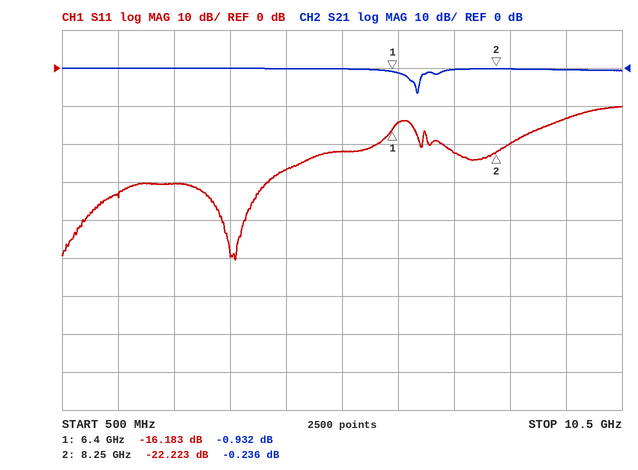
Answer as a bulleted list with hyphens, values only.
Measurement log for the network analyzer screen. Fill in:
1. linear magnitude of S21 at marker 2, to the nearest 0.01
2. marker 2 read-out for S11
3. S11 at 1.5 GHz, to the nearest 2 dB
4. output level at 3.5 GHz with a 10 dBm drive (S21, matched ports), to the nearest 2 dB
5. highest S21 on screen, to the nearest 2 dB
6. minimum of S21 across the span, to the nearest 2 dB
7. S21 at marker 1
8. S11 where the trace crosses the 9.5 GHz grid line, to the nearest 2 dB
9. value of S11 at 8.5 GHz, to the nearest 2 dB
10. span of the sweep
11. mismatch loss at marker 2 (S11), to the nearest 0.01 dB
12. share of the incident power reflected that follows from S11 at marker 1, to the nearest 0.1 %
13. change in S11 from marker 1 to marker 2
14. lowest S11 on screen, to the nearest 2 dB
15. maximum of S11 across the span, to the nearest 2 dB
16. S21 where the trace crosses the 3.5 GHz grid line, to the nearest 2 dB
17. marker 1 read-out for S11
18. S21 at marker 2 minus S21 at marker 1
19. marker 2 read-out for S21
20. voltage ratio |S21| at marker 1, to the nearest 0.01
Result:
- 0.97
- -22.223 dB
- -34 dB
- 10 dBm
- 0 dB
- -6 dB
- -0.932 dB
- -14 dB
- -20 dB
- 10 GHz
- 0.03 dB
- 2.4 %
- -6.040 dB
- -50 dB
- -10 dB
- 0 dB
- -16.183 dB
- 0.696 dB
- -0.236 dB
- 0.90
